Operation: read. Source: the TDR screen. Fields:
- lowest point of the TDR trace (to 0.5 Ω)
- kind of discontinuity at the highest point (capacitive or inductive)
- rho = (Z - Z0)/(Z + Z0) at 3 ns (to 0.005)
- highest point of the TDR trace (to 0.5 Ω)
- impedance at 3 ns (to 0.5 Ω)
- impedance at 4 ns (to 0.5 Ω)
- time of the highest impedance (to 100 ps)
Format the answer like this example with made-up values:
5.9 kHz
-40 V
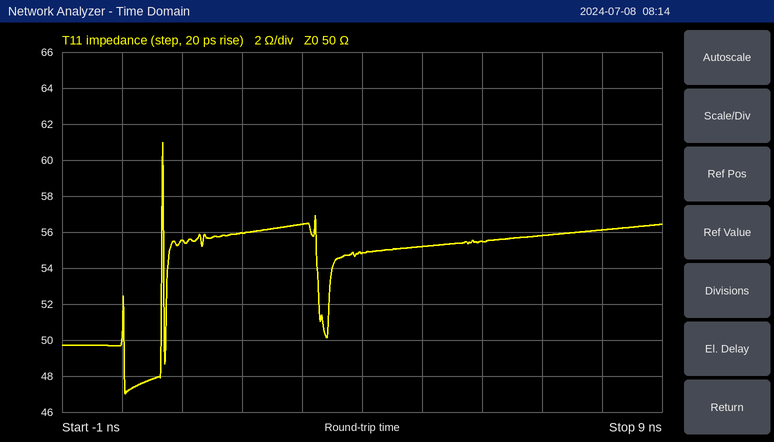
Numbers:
47.0 Ω
inductive
+0.060
61.0 Ω
56.5 Ω
55.0 Ω
700 ps
